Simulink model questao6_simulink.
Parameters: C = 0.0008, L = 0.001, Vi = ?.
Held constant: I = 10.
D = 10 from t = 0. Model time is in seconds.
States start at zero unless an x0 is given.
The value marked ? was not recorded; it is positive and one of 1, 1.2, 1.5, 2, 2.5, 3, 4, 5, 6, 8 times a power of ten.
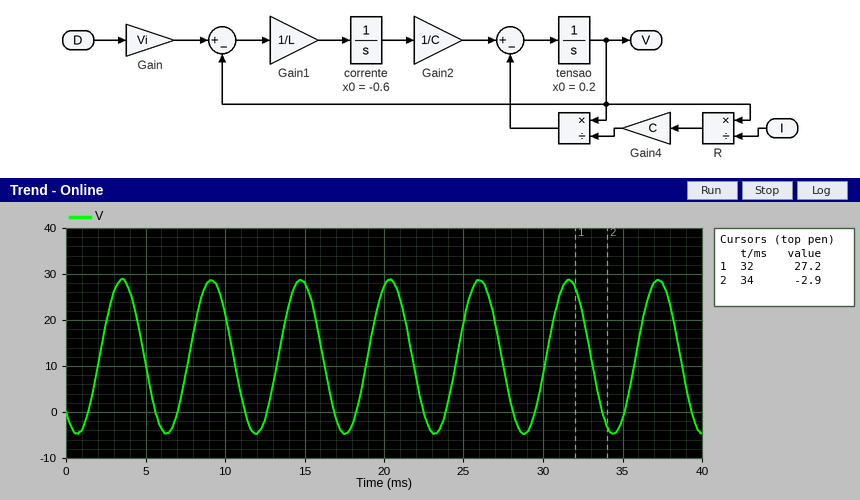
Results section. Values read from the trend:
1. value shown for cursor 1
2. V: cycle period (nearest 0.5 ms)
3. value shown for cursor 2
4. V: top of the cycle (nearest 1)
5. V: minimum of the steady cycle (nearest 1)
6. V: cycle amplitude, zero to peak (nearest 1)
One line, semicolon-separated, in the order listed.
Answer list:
27.2; 5.5 ms; -2.9; 29; -5; 17
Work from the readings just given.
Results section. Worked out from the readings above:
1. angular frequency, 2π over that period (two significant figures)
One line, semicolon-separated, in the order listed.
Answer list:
1.1 rad/ms
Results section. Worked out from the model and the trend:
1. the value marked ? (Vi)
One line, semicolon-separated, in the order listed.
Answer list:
1.2
